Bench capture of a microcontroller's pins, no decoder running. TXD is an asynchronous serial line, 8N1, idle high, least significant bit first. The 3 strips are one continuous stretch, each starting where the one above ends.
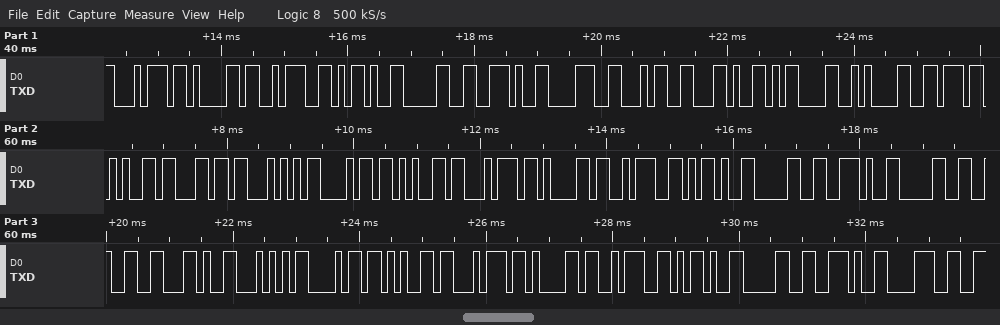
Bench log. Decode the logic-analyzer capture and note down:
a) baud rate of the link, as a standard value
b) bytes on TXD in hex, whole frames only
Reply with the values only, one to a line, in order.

9600 baud
74 61 3A 2D 30 2E 38 34 2C 0D 0A 76 65 6C 54 68 65 74 61 3A 2D 30 2E 30 32 2C 54 68 65 74 61 3A 2D 30 2E 38
